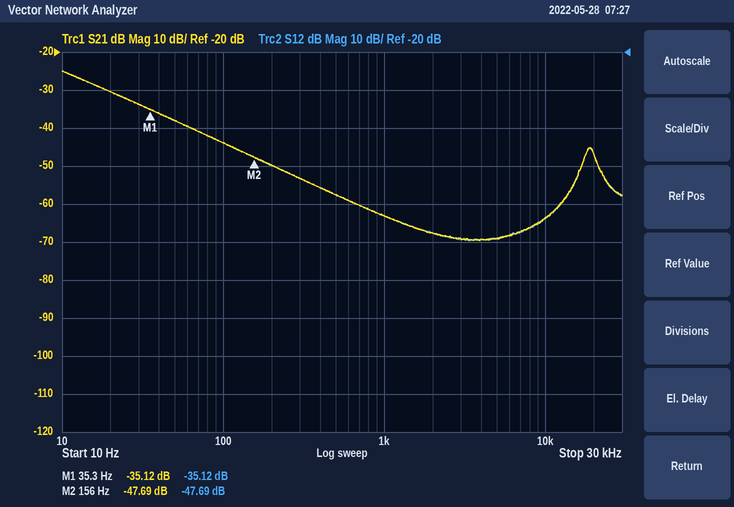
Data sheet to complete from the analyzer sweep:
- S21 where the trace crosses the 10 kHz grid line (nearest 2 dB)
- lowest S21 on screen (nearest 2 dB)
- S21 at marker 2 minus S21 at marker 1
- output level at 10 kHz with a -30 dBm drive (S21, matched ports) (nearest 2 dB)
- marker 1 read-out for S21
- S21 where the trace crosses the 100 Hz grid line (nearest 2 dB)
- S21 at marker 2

-64 dB
-70 dB
-12.57 dB
-94 dBm
-35.12 dB
-44 dB
-47.69 dB
